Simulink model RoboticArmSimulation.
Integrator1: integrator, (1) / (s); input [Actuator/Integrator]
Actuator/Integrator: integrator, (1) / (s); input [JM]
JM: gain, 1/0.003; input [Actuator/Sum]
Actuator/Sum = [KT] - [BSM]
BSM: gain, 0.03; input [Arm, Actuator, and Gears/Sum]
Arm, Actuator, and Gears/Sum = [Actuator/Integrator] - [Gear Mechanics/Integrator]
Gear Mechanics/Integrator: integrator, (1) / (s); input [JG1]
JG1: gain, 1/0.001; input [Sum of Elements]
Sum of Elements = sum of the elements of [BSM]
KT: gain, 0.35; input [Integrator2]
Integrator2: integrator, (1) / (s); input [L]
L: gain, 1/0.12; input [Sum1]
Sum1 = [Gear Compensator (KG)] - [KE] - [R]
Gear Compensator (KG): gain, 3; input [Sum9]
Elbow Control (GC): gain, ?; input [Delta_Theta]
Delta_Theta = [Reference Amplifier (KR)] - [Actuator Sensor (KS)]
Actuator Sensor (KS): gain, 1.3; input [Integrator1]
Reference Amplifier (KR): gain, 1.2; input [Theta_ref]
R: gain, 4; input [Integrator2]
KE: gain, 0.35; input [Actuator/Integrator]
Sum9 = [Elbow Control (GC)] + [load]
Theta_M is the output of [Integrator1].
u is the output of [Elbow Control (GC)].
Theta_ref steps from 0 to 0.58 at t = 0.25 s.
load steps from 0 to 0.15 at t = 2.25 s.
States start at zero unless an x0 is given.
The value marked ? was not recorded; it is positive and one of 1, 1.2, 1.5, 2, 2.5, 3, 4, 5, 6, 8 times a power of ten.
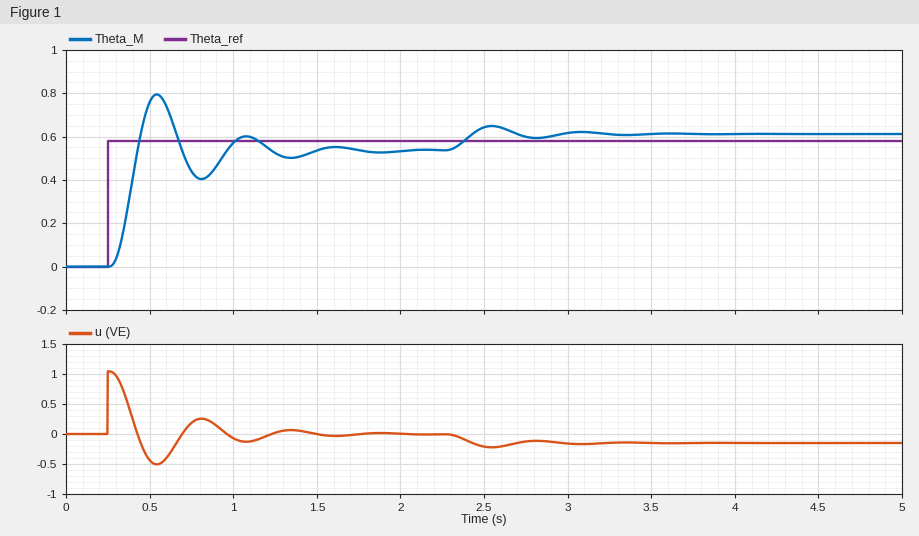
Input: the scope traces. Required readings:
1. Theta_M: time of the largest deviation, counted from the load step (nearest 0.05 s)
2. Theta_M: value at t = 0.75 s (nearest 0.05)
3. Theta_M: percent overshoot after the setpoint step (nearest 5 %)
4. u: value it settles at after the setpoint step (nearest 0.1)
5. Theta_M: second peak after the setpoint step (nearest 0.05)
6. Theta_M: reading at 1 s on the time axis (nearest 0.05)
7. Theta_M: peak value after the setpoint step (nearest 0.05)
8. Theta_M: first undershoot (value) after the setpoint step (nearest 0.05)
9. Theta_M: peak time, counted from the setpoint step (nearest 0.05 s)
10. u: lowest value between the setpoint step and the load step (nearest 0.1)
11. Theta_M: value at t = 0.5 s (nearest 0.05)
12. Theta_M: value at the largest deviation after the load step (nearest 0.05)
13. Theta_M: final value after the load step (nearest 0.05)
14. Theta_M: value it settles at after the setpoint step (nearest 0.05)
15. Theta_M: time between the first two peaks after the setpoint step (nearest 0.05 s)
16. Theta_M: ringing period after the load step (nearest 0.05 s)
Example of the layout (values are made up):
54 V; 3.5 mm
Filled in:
0.30 s; 0.45; 50 %; 0.0; 0.60; 0.55; 0.80; 0.40; 0.30 s; -0.5; 0.75; 0.65; 0.60; 0.55; 0.55 s; 0.55 s
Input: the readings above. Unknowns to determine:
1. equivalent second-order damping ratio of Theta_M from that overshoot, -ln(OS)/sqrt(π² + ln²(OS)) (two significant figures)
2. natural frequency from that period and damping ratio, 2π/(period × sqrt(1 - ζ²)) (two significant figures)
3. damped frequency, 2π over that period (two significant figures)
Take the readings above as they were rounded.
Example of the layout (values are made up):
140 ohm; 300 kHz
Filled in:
0.22; 12 rad/s; 11 rad/s
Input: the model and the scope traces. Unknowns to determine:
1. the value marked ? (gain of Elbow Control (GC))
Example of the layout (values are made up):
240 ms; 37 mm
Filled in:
1.5
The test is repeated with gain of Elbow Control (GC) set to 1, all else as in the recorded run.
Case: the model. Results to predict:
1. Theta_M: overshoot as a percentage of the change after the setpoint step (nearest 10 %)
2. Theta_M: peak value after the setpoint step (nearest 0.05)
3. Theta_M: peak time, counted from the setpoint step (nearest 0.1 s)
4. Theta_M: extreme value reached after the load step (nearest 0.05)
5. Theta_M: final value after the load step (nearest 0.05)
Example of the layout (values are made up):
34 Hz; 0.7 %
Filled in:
30 %; 0.70; 0.4 s; 0.70; 0.65
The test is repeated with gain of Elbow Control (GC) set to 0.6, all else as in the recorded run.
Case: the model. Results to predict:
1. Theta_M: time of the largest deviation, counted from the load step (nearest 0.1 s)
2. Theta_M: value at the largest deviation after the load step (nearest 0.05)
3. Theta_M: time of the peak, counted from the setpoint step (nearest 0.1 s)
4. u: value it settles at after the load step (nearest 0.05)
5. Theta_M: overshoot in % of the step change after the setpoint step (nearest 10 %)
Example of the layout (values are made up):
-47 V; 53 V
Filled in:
0.5 s; 0.75; 0.5 s; -0.15; 20 %
